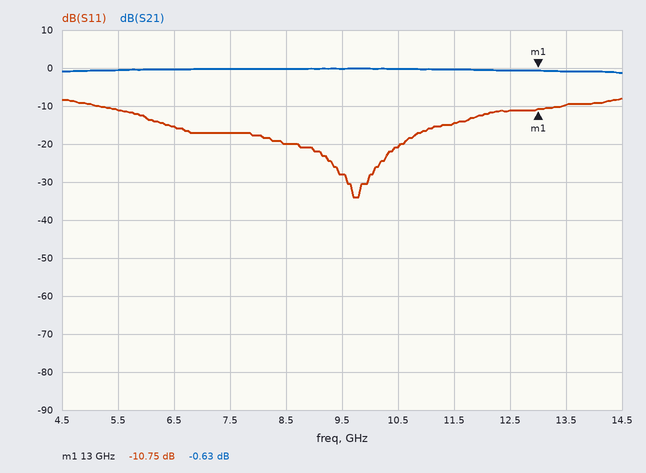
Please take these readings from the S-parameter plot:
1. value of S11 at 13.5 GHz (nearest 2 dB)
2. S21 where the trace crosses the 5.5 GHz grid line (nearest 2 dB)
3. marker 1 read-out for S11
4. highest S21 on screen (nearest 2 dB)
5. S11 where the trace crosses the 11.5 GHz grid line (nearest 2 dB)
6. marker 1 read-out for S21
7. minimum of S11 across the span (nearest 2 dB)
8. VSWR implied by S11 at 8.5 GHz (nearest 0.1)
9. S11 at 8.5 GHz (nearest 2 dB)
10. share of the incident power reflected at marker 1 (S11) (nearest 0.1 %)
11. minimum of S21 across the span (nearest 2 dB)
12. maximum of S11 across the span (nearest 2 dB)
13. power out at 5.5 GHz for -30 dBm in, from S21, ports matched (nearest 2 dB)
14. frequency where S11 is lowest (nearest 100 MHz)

-10 dB
0 dB
-10.75 dB
0 dB
-14 dB
-0.63 dB
-34 dB
1.2
-20 dB
8.4 %
-2 dB
-8 dB
-30 dBm
9.7 GHz
